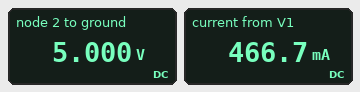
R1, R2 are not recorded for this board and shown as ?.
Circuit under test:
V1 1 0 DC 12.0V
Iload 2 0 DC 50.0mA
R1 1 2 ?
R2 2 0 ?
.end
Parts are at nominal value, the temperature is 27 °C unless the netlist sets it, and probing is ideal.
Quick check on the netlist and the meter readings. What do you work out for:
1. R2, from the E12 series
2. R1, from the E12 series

12 Ω
15 Ω
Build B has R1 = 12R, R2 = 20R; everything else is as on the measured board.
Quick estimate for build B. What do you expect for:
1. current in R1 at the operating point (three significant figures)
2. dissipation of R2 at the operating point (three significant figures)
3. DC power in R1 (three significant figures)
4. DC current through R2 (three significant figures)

406 mA
2.54 W
1.98 W
356 mA
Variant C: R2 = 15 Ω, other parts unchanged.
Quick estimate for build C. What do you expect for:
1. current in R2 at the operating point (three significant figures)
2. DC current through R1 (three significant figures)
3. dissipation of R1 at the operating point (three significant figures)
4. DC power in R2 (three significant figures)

375 mA
425 mA
2.71 W
2.11 W
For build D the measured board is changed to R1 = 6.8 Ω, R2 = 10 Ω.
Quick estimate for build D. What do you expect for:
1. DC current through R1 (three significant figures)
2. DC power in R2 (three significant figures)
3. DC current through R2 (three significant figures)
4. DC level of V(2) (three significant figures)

744 mA
4.82 W
694 mA
6.94 V
